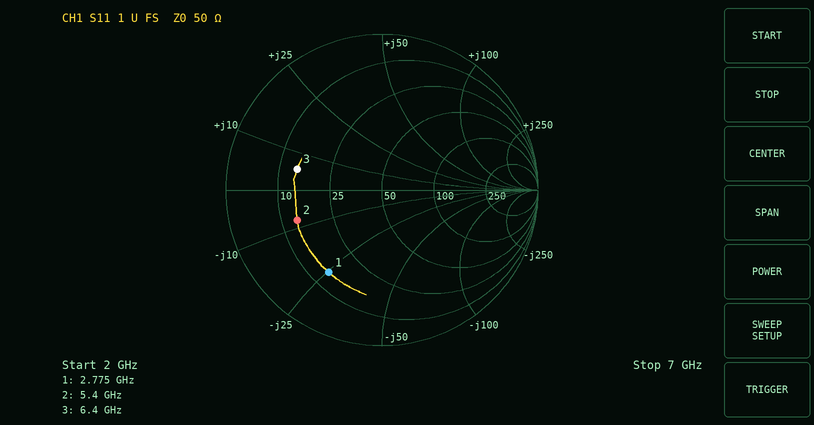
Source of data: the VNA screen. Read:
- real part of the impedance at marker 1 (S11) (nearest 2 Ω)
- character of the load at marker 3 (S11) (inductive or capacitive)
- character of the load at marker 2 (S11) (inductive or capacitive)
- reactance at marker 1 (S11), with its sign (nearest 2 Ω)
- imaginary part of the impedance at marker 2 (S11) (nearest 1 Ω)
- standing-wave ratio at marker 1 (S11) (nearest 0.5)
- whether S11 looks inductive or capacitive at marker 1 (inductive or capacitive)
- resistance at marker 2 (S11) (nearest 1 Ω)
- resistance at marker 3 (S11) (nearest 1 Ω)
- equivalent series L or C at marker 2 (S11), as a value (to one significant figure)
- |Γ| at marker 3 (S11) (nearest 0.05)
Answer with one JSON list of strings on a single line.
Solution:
["14 Ω", "inductive", "capacitive", "-26 Ω", "-8 Ω", "4.5", "capacitive", "14 Ω", "14 Ω", "4 pF", "0.55"]
